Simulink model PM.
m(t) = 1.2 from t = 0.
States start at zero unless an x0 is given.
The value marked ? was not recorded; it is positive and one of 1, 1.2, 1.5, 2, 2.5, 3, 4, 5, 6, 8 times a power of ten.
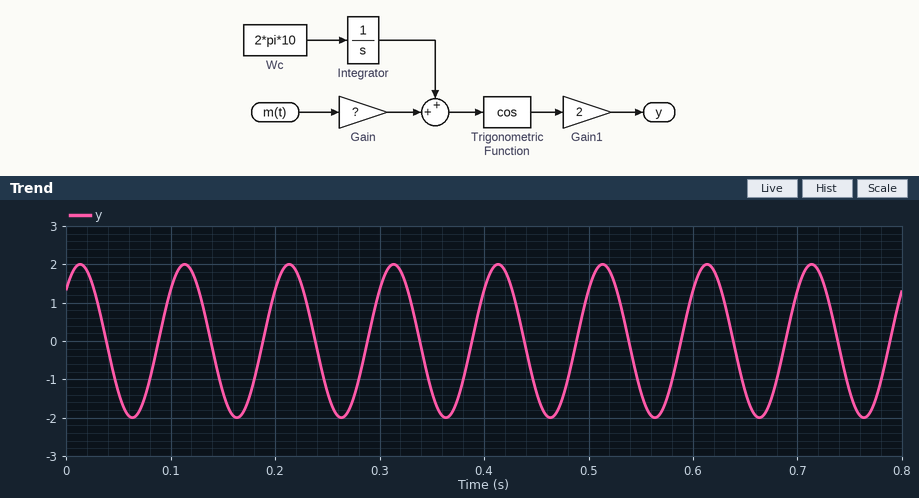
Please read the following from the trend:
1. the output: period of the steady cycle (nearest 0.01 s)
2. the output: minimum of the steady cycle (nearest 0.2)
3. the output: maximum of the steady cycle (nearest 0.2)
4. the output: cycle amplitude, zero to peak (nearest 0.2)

0.10 s
-2.0
2.0
2.0
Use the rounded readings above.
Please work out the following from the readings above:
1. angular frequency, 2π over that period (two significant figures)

63 rad/s
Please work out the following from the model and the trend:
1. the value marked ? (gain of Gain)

15
